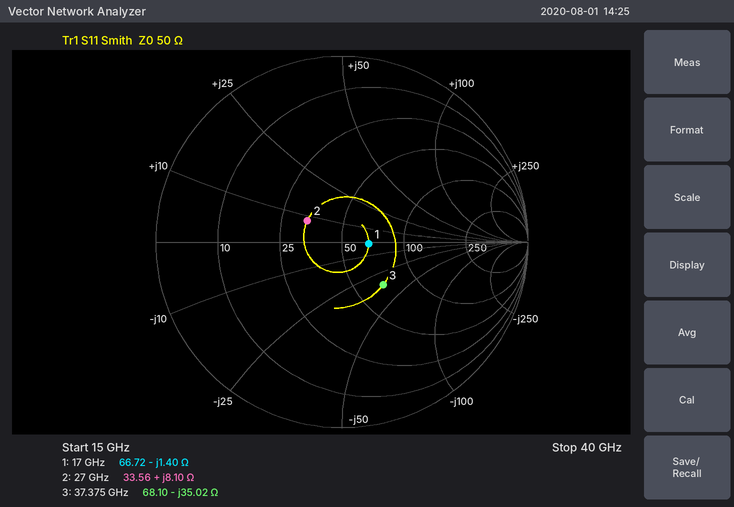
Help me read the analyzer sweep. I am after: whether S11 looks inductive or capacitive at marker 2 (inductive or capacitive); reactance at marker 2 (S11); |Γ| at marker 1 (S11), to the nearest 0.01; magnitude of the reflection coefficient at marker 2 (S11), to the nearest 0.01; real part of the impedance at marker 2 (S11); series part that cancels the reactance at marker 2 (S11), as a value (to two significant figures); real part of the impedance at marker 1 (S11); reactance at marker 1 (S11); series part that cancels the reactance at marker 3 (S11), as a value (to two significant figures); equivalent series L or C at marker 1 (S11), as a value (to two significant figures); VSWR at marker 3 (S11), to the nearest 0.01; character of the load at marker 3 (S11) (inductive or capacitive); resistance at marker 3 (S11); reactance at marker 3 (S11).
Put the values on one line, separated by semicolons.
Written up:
inductive; +8.10 Ω; 0.14; 0.22; 33.56 Ω; 730 fF; 66.72 Ω; -1.40 Ω; 150 pH; 6.7 pF; 1.94; capacitive; 68.10 Ω; -35.02 Ω
